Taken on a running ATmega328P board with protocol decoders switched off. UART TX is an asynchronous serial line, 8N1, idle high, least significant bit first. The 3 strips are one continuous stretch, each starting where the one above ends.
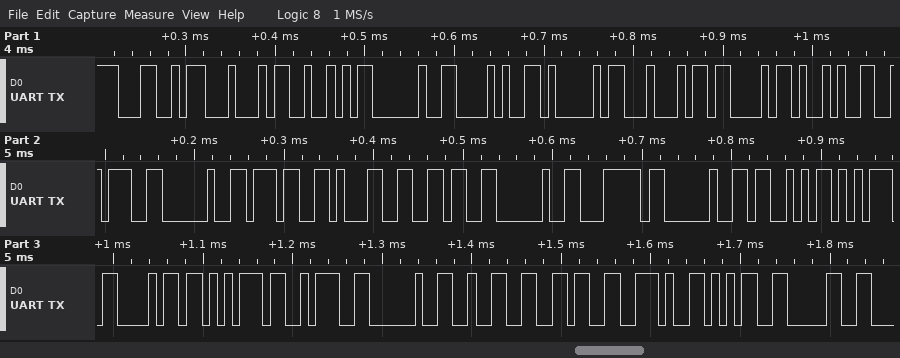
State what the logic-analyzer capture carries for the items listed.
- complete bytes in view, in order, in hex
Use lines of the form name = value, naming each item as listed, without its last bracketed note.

complete bytes in view, in order, in hex = 4C 44 52 20 28 41 44 43 29 3A 20 37 31 36 20 7C 20 53 75 68 75 3A 20 32 36 2E 35 30
